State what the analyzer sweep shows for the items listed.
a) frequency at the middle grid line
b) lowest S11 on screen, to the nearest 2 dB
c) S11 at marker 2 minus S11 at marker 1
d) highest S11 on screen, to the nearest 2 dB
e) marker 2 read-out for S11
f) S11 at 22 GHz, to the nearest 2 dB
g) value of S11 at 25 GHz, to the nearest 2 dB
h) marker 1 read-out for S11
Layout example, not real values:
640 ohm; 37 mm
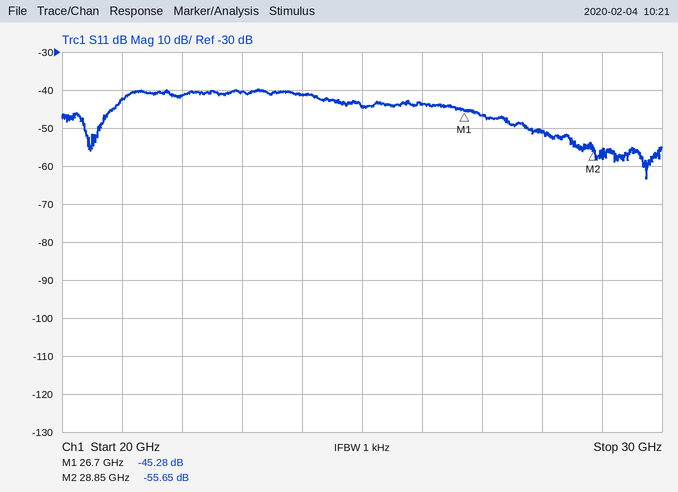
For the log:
25 GHz; -64 dB; -10.37 dB; -40 dB; -55.65 dB; -42 dB; -44 dB; -45.28 dB
